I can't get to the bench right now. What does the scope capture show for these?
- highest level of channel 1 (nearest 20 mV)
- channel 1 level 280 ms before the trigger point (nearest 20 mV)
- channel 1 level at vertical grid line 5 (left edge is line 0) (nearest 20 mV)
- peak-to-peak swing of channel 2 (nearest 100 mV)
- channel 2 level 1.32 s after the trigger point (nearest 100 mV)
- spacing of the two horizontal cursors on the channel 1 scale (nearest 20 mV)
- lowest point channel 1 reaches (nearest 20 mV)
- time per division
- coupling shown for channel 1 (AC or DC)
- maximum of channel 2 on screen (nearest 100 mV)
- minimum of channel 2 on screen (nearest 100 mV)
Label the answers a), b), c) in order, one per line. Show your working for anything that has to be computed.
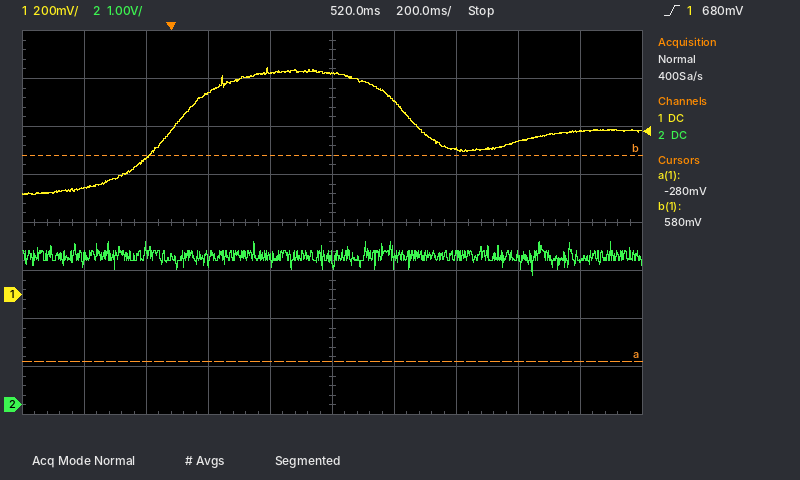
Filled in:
a) 940 mV
b) 440 mV
c) 920 mV
d) 3.4 V − (2.7 V) = 700 mV
e) 3.0 V
f) 860 mV
g) 420 mV
h) 200 ms
i) DC
j) 3.4 V
k) 2.7 V
